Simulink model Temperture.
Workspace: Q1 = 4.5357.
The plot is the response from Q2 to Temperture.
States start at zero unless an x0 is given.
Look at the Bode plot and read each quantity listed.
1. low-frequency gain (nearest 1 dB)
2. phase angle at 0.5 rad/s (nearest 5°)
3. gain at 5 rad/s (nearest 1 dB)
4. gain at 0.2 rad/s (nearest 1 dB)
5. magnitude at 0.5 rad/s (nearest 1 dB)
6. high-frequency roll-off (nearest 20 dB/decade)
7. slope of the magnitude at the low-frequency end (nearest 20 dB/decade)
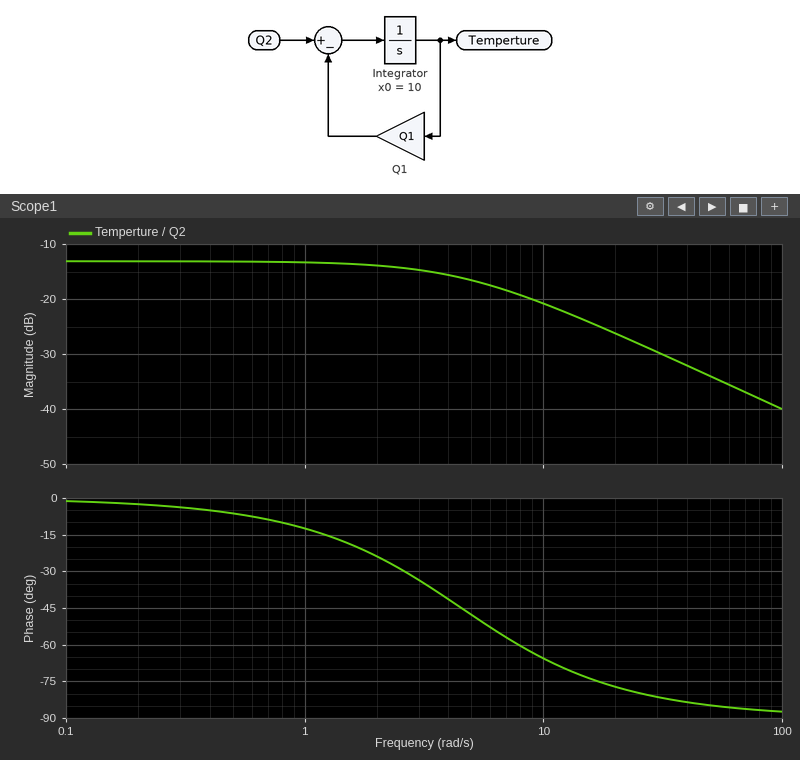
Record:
-13 dB
-5°
-17 dB
-13 dB
-13 dB
-20 dB/decade
0 dB/decade
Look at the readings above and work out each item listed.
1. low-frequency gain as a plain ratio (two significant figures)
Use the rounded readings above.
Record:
0.22
